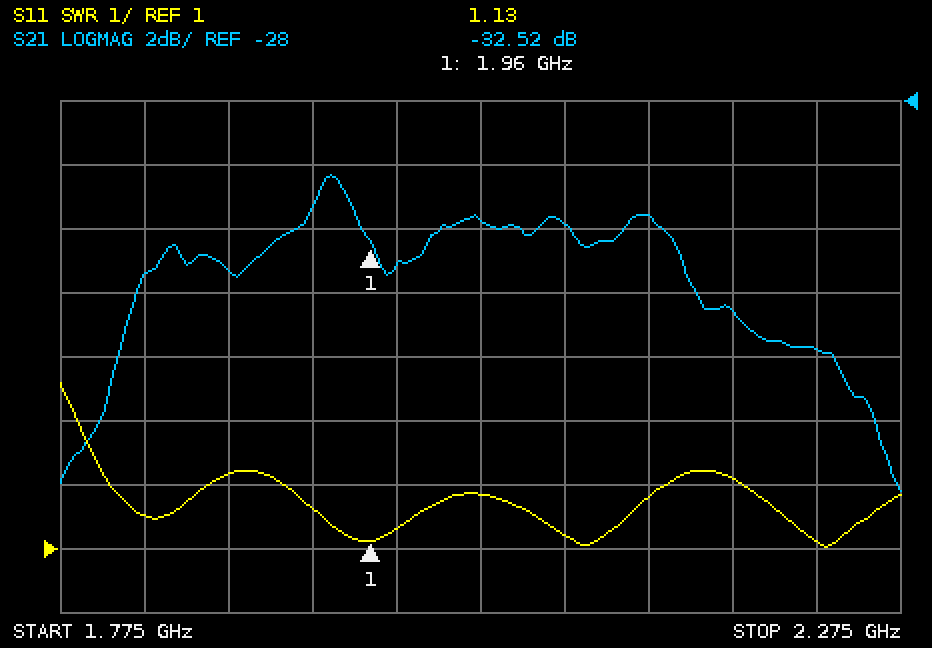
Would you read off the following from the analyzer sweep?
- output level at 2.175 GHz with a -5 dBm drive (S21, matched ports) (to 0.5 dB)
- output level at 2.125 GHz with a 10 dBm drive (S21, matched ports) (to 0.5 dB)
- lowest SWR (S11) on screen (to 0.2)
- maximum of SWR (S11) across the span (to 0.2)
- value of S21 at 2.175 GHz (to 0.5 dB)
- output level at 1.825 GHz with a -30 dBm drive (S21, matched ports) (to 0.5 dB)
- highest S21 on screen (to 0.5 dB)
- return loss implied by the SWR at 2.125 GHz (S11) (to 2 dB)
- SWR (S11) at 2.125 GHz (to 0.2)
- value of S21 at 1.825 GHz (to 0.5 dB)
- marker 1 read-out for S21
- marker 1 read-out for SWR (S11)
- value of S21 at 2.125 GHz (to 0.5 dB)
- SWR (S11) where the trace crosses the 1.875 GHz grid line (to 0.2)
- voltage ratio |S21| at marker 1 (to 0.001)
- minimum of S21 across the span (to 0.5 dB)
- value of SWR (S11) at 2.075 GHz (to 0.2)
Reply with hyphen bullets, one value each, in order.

- -39.5 dBm
- -21.5 dBm
- 1.0
- 3.6
- -34.5 dB
- -63.5 dBm
- -30.5 dB
- 10 dB
- 1.8
- -33.5 dB
- -32.52 dB
- 1.13
- -31.5 dB
- 2.2
- 0.024
- -40.0 dB
- 1.2
